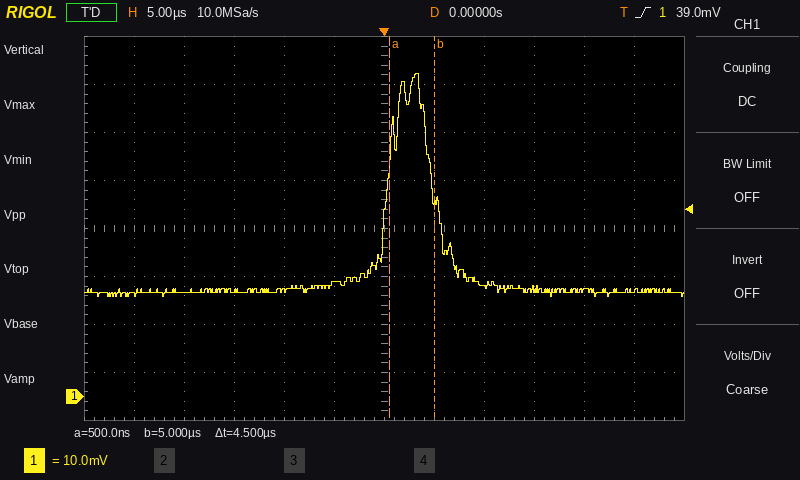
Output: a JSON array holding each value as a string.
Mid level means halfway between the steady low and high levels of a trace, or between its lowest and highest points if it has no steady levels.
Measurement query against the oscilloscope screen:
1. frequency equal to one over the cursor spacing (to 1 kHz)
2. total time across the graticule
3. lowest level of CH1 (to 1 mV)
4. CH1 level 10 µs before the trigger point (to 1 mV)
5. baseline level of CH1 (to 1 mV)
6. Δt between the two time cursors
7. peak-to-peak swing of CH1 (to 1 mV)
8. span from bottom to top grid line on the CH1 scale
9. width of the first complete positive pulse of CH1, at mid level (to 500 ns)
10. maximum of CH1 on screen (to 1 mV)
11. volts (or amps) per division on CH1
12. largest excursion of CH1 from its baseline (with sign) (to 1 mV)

["222 kHz", "60 µs", "21 mV", "22 mV", "22 mV", "4.5 µs", "46 mV", "80 mV", "4.5 µs", "67 mV", "10 mV", "+45 mV"]
